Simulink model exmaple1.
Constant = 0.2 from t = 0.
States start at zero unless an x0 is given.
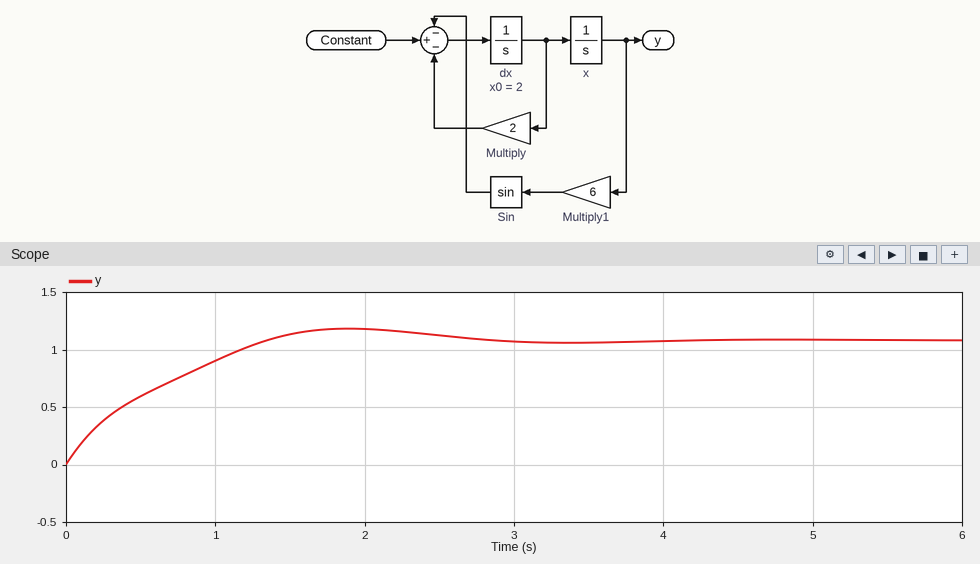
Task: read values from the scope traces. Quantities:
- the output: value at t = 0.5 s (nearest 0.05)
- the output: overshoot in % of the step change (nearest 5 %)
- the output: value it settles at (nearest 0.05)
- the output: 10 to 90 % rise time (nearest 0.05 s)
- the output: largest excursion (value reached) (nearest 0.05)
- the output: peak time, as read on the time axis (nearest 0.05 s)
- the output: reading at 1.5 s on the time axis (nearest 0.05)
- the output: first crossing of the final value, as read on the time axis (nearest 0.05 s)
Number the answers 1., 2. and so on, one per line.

1. 0.60
2. 10 %
3. 1.10
4. 1.05 s
5. 1.20
6. 1.90 s
7. 1.15
8. 1.35 s
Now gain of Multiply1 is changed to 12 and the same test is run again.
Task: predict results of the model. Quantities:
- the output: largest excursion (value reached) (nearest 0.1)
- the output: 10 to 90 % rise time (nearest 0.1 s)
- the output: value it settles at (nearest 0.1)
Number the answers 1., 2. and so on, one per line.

1. 1.1
2. 1.2 s
3. 1.1
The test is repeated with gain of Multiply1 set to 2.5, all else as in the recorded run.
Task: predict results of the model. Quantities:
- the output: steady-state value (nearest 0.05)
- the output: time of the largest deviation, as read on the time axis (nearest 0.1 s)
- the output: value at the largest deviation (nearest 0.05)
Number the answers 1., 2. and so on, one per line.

1. 0.10
2. 0.9 s
3. 0.70
